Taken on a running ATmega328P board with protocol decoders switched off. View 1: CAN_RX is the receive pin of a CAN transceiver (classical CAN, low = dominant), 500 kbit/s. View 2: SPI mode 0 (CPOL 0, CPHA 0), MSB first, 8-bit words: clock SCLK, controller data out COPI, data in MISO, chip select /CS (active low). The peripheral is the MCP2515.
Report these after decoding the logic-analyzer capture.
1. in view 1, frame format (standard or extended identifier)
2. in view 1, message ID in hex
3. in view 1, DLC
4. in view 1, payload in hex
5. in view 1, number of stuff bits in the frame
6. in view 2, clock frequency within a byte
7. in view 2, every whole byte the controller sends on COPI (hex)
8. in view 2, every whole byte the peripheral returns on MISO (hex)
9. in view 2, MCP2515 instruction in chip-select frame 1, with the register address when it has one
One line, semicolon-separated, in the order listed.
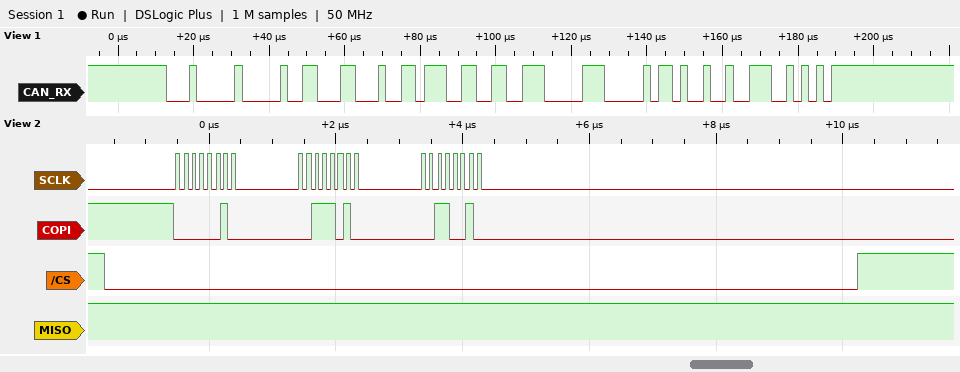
standard; 0x100; 6; 31 37 33 38 30 34; 4; 8 MHz; 02 3A 32; FF FF FF; WRITE 0x3A
